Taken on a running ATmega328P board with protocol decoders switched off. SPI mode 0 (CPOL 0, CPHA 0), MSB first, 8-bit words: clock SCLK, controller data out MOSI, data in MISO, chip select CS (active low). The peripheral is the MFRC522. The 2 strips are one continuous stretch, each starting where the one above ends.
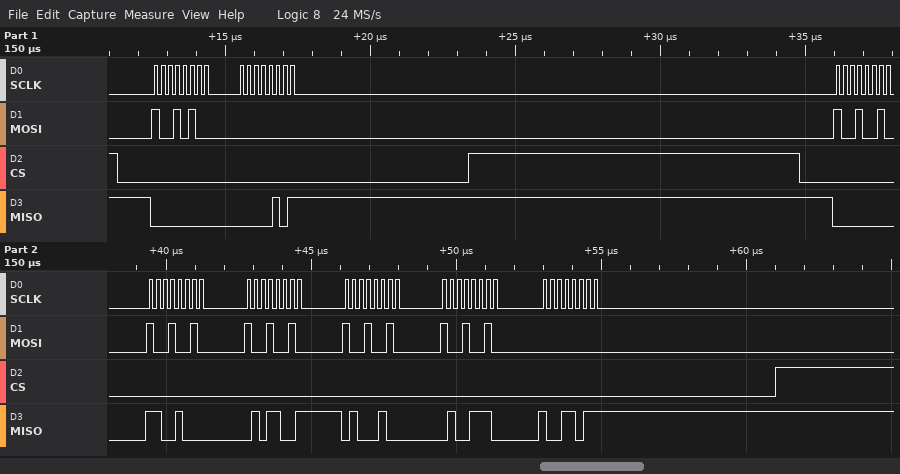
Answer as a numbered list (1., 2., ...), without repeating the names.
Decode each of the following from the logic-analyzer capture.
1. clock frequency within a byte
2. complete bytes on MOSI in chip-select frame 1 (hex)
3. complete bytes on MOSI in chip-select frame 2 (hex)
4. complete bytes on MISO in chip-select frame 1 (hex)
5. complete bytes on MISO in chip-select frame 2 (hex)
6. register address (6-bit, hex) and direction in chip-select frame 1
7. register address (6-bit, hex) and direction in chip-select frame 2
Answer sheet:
1. 4 MHz
2. 94 00
3. 92 92 92 92 92 00
4. 00 05
5. 00 C8 59 44 4E 9B
6. 0x0A read
7. 0x09 read
